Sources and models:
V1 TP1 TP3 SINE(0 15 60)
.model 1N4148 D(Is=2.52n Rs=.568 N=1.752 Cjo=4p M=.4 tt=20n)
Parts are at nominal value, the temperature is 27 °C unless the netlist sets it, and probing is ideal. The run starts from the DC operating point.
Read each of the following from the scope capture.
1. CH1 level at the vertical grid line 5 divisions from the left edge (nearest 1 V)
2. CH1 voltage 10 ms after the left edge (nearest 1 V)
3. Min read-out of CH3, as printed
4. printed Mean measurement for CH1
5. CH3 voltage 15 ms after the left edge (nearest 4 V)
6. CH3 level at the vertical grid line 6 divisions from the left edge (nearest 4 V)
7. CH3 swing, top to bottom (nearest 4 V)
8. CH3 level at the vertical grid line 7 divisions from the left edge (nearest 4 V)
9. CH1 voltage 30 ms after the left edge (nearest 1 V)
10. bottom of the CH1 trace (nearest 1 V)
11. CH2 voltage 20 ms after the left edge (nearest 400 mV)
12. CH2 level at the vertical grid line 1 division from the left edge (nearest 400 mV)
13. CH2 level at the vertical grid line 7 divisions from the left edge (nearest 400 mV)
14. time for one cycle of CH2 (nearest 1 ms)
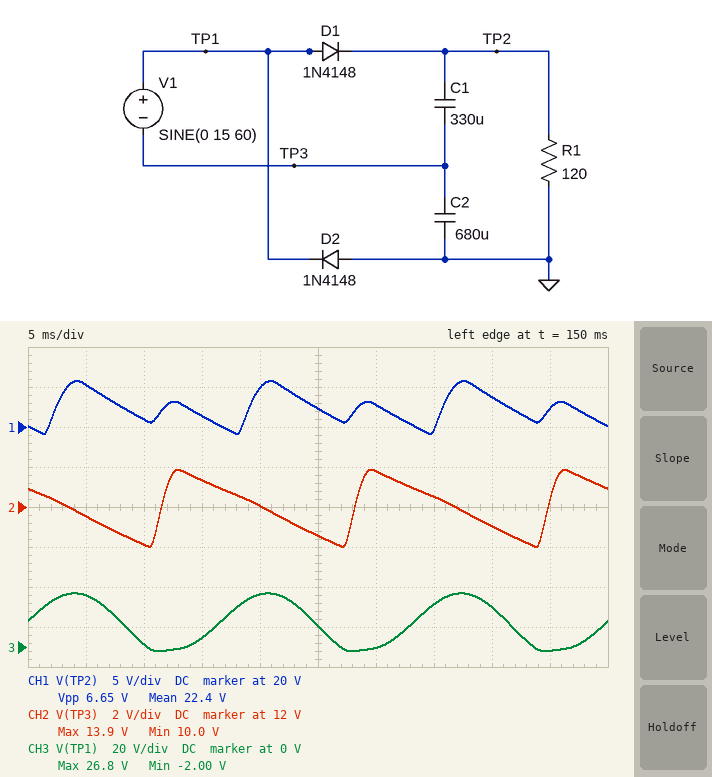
22 V
21 V
-2.00 V
22.4 V
4 V
0 V
28 V
20 V
23 V
19 V
12.0 V
11.6 V
12.4 V
17 ms
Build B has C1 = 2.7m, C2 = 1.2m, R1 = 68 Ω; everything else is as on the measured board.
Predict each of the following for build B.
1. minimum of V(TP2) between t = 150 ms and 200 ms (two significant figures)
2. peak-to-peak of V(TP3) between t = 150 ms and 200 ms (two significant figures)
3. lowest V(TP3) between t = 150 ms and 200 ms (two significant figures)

22 V
4.0 V
9.5 V
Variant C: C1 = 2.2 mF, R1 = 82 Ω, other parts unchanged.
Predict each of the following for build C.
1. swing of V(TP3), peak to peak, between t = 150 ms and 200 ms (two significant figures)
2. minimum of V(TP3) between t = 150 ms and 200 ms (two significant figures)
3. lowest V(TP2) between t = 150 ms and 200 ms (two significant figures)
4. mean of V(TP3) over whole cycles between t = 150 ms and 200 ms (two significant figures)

5.7 V
8.1 V
21 V
11 V
